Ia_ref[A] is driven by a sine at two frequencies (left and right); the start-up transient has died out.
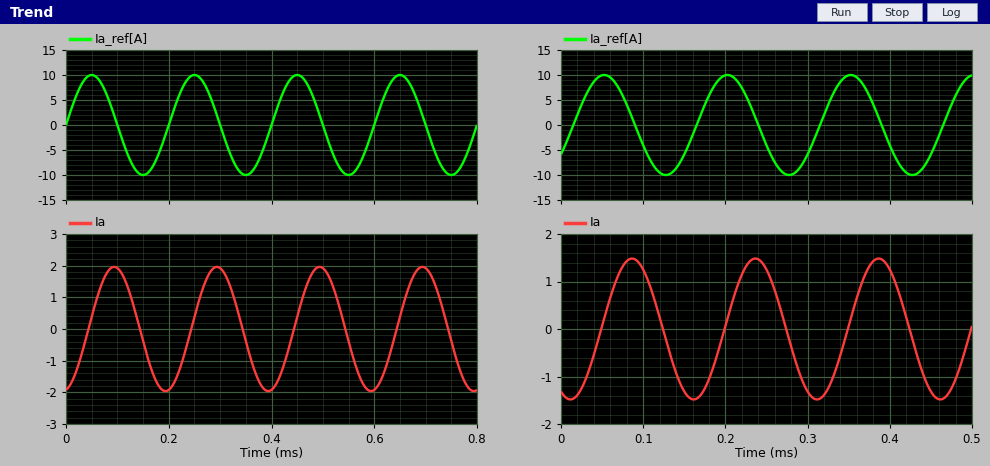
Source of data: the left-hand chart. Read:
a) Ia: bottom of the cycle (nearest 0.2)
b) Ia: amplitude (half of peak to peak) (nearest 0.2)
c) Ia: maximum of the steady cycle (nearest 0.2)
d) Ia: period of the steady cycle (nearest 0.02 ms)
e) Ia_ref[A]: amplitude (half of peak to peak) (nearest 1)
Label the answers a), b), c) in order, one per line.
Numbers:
a) -2.0
b) 2.0
c) 2.0
d) 0.20 ms
e) 10
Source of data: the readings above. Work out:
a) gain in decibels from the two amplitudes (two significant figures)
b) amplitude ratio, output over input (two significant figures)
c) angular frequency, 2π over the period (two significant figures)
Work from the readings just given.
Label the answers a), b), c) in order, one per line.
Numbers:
a) -14 dB
b) 0.20
c) 31 rad/ms
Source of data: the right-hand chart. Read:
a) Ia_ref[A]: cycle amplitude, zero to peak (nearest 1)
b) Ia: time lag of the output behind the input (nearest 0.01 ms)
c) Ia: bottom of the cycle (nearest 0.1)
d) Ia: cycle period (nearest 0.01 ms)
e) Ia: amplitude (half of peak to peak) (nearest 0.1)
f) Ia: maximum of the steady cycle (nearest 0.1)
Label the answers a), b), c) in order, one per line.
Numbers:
a) 10
b) 0.03 ms
c) -1.5
d) 0.15 ms
e) 1.5
f) 1.5
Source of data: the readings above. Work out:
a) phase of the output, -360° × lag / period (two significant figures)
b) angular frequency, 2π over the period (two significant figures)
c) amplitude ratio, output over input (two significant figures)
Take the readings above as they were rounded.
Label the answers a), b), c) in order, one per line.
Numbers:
a) -72°
b) 42 rad/ms
c) 0.15
